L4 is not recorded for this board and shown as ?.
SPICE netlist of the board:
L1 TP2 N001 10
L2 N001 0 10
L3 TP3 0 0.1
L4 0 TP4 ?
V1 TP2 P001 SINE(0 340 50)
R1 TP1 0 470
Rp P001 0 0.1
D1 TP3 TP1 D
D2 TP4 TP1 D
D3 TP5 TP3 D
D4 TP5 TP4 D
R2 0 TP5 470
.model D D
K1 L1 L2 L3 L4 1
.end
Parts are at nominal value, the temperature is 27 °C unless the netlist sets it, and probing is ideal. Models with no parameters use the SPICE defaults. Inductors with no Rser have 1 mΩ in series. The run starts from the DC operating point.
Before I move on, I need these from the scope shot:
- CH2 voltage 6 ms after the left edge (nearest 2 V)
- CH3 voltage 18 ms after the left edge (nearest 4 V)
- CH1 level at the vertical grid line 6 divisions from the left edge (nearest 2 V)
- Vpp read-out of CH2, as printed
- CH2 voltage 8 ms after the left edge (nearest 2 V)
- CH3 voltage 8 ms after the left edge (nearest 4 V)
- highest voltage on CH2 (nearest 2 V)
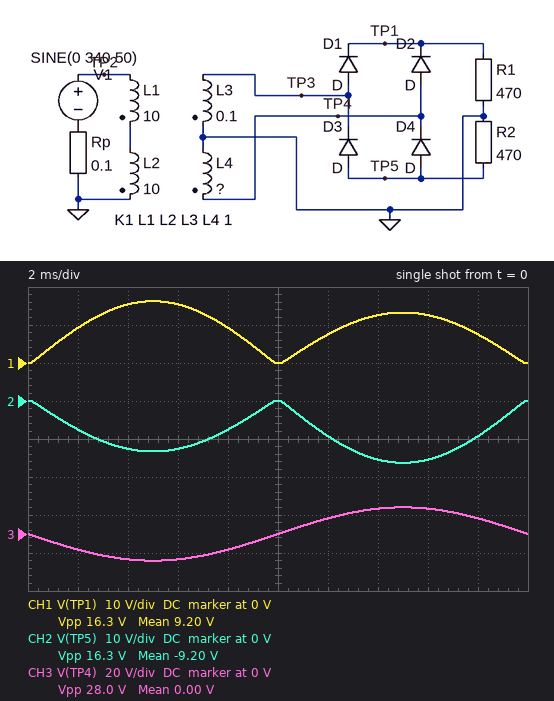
-12 V
8 V
8 V
16.3 V
-8 V
-8 V
0 V
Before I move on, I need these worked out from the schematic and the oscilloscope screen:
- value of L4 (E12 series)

68 mH
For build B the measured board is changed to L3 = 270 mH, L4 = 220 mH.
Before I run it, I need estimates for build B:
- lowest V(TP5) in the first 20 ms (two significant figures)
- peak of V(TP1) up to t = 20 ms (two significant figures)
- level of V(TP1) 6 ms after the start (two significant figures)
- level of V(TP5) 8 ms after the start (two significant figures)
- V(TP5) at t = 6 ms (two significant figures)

-27 V
27 V
26 V
-14 V
-23 V
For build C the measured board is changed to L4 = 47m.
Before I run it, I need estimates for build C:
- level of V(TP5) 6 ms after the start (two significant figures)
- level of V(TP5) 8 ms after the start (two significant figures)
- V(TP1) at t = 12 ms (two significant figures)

-10 V
-6.1 V
6.1 V
